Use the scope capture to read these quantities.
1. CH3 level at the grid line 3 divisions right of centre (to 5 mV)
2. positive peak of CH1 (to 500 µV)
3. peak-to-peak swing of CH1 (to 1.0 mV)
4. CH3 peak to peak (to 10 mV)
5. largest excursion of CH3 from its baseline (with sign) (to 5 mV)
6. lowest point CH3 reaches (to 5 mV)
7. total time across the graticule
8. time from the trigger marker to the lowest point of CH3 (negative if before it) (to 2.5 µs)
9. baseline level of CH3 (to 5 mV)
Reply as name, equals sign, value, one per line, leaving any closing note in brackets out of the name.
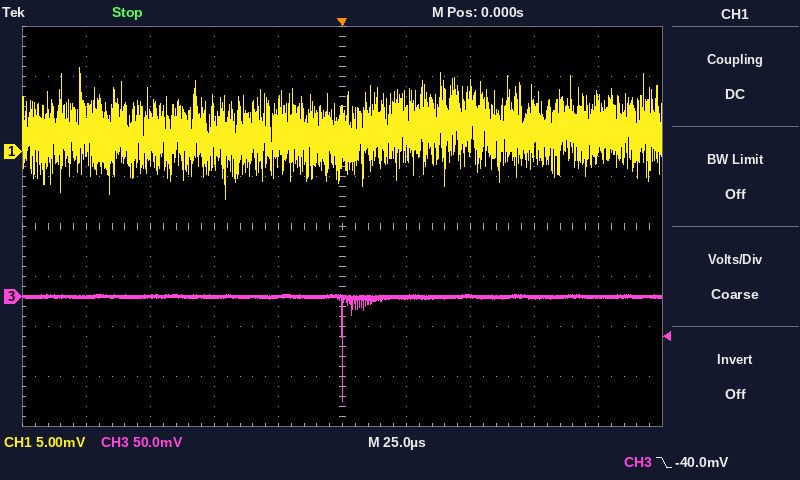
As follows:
CH3 level at the grid line 3 divisions right of centre = 0 mV
positive peak of CH1 = 8.5 mV
peak-to-peak swing of CH1 = 13.0 mV
CH3 peak to peak = 110 mV
largest excursion of CH3 from its baseline (with sign) = -105 mV
lowest point CH3 reaches = -105 mV
total time across the graticule = 250 µs
time from the trigger marker to the lowest point of CH3 (negative if before it) = 0.0 µs
baseline level of CH3 = 0 mV
